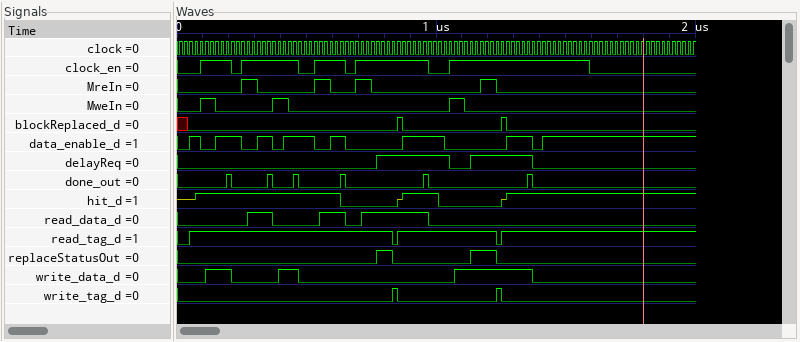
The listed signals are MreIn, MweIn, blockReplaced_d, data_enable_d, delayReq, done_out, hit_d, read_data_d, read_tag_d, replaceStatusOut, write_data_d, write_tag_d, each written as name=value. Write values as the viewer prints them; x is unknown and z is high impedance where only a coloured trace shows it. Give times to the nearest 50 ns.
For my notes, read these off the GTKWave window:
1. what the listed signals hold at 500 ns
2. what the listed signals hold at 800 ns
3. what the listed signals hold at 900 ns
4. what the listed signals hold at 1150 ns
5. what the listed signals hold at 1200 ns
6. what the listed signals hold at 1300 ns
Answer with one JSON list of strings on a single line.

["MreIn=0, MweIn=0, blockReplaced_d=0, data_enable_d=1, delayReq=0, done_out=0, hit_d=1, read_data_d=0, read_tag_d=1, replaceStatusOut=0, write_data_d=0, write_tag_d=0", "MreIn=0, MweIn=0, blockReplaced_d=0, data_enable_d=0, delayReq=1, done_out=0, hit_d=0, read_data_d=1, read_tag_d=1, replaceStatusOut=1, write_data_d=0, write_tag_d=0", "MreIn=0, MweIn=0, blockReplaced_d=0, data_enable_d=1, delayReq=1, done_out=0, hit_d=1, read_data_d=1, read_tag_d=1, replaceStatusOut=0, write_data_d=0, write_tag_d=0", "MreIn=0, MweIn=0, blockReplaced_d=0, data_enable_d=0, delayReq=1, done_out=0, hit_d=0, read_data_d=0, read_tag_d=1, replaceStatusOut=1, write_data_d=1, write_tag_d=0", "MreIn=1, MweIn=0, blockReplaced_d=0, data_enable_d=0, delayReq=1, done_out=0, hit_d=0, read_data_d=0, read_tag_d=1, replaceStatusOut=1, write_data_d=1, write_tag_d=0", "MreIn=0, MweIn=0, blockReplaced_d=0, data_enable_d=1, delayReq=1, done_out=0, hit_d=1, read_data_d=0, read_tag_d=1, replaceStatusOut=0, write_data_d=1, write_tag_d=0"]
